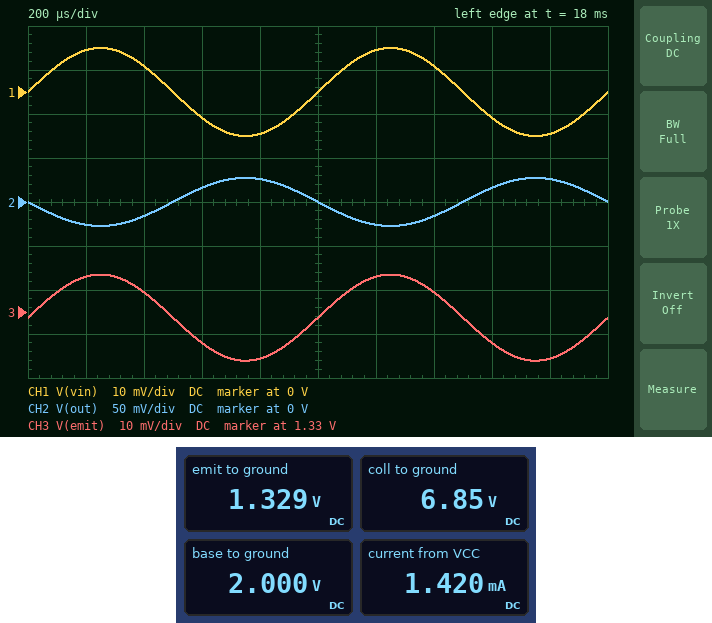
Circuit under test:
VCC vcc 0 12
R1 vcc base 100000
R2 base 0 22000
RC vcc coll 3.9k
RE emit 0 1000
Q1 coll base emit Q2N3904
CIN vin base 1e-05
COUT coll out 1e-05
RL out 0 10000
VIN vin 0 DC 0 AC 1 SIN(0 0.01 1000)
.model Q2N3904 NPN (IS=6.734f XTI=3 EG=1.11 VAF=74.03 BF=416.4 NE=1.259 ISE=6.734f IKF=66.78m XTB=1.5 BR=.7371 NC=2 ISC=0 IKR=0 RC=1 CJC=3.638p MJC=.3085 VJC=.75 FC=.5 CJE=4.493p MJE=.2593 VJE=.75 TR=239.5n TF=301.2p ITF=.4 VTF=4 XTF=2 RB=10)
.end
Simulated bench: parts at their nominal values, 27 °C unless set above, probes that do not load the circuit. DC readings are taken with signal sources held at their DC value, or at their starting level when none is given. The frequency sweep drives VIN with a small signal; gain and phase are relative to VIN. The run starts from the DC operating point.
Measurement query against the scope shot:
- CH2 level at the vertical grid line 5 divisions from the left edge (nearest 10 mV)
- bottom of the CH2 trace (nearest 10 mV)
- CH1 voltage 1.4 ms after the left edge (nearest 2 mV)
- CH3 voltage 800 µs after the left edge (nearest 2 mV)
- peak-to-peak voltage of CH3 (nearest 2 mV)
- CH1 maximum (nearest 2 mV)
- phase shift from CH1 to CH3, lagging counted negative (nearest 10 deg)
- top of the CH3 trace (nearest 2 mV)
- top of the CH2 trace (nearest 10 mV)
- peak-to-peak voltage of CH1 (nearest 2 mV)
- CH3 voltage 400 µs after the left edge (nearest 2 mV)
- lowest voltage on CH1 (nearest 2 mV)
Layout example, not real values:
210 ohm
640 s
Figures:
0 V
-30 mV
6 mV
1.320 V
20 mV
10 mV
0 deg
1.338 V
30 mV
20 mV
1.334 V
-10 mV
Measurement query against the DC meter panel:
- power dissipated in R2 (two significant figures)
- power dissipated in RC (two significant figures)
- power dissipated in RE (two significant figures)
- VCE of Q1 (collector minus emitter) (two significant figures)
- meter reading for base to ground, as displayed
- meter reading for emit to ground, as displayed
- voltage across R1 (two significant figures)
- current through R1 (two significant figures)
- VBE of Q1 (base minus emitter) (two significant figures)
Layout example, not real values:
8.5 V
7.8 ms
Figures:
180 µW
6.8 mW
1.8 mW
5.5 V
2.000 V
1.329 V
10 V
100 µA
670 mV
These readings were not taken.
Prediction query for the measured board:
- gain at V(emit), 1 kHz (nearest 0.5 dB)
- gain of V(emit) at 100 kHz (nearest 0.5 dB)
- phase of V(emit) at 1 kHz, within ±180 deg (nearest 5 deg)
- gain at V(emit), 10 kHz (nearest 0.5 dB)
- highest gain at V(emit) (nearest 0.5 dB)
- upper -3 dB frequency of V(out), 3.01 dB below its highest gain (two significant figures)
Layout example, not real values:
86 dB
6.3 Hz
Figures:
0 dB
0 dB
0 deg
0 dB
0 dB
36 MHz
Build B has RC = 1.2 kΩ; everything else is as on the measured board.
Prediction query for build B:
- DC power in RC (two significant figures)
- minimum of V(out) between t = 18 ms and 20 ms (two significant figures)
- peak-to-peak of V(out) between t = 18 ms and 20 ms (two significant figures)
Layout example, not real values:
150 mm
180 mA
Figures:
2.1 mW
-10 mV
21 mV
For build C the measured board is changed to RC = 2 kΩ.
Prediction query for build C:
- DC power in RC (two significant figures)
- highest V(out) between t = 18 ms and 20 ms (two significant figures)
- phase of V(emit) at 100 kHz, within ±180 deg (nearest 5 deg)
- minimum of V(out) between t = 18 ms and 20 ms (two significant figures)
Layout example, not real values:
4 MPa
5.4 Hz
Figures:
3.5 mW
16 mV
0 deg
-16 mV
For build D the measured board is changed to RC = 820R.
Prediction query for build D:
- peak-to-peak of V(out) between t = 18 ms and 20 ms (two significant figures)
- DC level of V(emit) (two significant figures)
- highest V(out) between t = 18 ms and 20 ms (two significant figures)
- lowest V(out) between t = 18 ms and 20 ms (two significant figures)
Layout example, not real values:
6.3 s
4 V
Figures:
15 mV
1.3 V
7.4 mV
-7.4 mV
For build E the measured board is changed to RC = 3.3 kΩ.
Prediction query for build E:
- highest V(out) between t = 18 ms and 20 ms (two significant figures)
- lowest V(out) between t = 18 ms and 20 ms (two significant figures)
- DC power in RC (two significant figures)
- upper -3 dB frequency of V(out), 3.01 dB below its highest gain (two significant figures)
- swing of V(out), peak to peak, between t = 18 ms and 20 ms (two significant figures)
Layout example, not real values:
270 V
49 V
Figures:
24 mV
-24 mV
5.8 mW
46 MHz
48 mV
